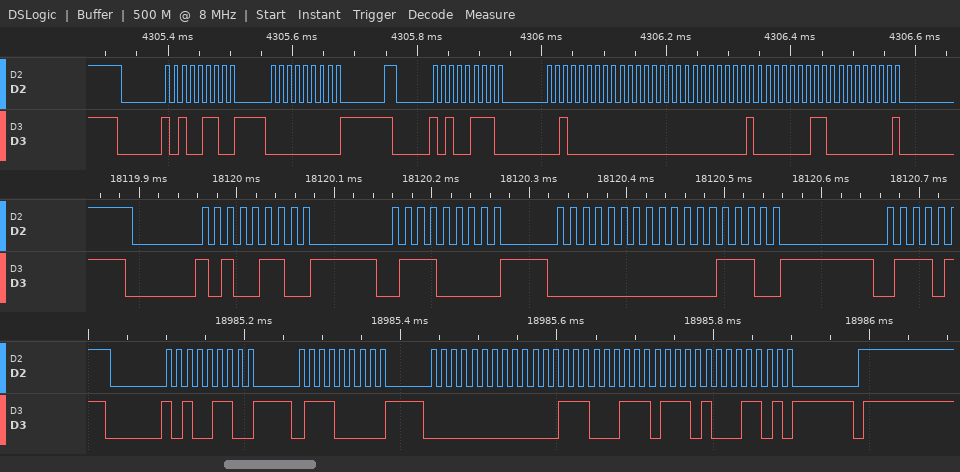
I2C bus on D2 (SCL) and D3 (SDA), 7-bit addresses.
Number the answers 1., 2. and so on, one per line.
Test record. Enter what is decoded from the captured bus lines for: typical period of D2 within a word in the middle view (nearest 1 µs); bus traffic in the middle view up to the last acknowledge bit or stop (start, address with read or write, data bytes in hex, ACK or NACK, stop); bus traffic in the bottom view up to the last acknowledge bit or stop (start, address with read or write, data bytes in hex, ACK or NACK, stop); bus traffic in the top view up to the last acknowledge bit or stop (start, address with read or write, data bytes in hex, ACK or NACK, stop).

1. 13 µs
2. start, address 53 write ACK, 70 ACK, 00 ACK, 0E ACK
3. start, address 53 write ACK, 70 ACK, 00 ACK, 0E ACK, 77 ACK, 8D ACK, stop
4. start, address 53 write ACK, 00 ACK, repeated start, address 53 read ACK, 20 ACK, 00 ACK, 01 ACK, 03 ACK
